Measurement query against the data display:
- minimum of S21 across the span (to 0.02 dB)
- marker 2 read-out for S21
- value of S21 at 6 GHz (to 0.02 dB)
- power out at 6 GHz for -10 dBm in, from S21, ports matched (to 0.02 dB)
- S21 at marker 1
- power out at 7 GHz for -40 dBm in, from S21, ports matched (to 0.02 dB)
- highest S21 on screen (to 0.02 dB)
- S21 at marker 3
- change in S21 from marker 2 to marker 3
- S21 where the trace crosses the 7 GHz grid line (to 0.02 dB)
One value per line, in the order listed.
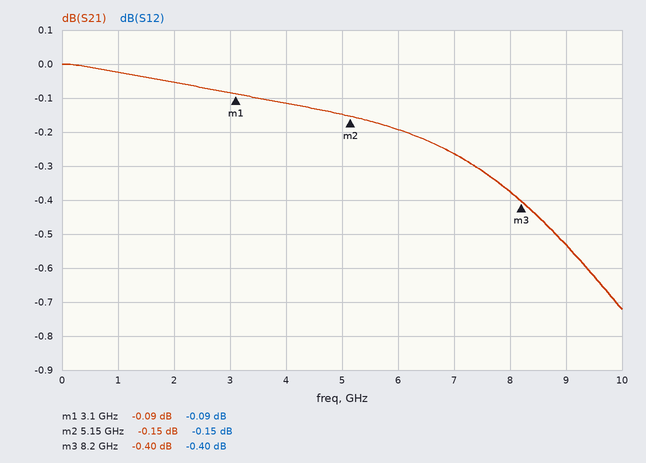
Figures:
-0.72 dB
-0.15 dB
-0.20 dB
-10.20 dBm
-0.09 dB
-40.26 dBm
0.00 dB
-0.40 dB
-0.25 dB
-0.26 dB
